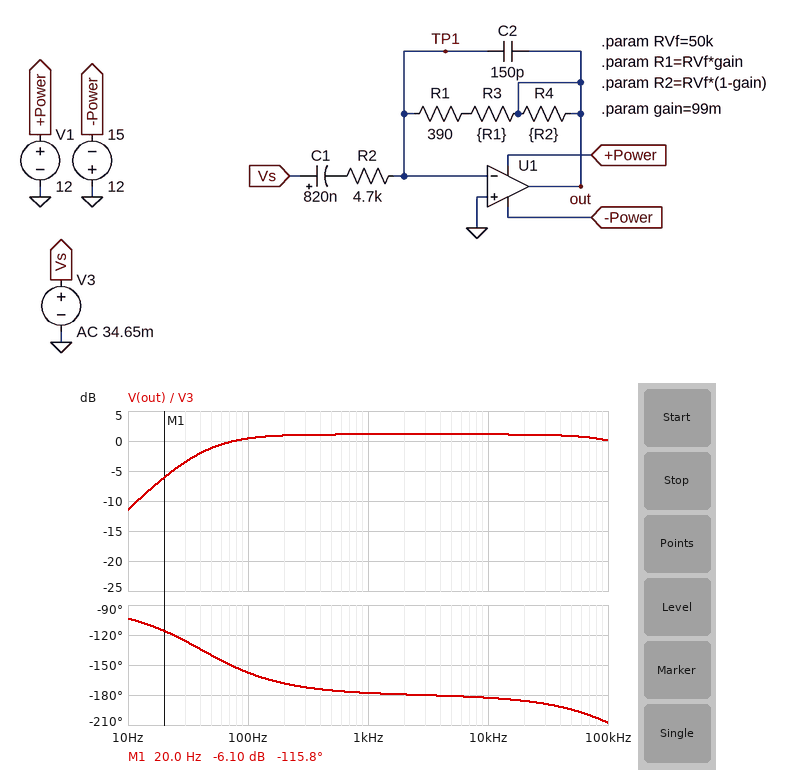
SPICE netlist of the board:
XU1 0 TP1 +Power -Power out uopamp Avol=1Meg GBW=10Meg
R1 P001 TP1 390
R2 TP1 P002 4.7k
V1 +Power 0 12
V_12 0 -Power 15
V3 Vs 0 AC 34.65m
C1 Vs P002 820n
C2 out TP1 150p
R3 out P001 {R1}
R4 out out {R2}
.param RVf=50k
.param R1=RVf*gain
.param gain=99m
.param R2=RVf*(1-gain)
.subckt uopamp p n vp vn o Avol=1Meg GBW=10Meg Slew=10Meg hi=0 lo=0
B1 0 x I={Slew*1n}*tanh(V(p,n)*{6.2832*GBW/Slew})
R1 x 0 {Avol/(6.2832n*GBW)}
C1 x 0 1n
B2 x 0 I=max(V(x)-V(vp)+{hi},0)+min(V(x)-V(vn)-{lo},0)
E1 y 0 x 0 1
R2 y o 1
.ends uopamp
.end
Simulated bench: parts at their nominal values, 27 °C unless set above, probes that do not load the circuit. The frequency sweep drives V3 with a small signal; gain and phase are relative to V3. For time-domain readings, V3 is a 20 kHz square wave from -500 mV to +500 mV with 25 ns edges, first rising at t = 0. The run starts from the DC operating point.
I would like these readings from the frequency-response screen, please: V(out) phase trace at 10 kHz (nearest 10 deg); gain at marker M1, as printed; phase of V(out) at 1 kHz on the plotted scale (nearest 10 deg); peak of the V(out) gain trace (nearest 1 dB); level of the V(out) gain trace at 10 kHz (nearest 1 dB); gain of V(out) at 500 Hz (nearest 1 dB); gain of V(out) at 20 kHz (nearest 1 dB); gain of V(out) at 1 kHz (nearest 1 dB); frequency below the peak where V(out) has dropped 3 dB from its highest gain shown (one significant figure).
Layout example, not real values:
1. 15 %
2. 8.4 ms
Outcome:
1. -180 deg
2. -6.10 dB
3. -180 deg
4. 1 dB
5. 1 dB
6. 1 dB
7. 1 dB
8. 1 dB
9. 40 Hz
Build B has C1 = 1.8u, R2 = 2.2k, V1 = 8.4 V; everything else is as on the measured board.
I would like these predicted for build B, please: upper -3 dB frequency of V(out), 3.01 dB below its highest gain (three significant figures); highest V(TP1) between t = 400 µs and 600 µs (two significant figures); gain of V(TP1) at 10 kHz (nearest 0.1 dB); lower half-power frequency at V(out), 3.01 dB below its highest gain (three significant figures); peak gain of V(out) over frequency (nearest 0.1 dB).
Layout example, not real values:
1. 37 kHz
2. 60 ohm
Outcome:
1. 189 kHz
2. 44 mV
3. -52.3 dB
4. 40.2 Hz
5. 7.7 dB
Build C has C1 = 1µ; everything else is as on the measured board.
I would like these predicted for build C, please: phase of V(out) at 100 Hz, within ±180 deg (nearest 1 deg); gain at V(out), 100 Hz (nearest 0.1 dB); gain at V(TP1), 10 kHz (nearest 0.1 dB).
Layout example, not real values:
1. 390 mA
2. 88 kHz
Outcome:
1. -161 deg
2. 0.6 dB
3. -58.9 dB
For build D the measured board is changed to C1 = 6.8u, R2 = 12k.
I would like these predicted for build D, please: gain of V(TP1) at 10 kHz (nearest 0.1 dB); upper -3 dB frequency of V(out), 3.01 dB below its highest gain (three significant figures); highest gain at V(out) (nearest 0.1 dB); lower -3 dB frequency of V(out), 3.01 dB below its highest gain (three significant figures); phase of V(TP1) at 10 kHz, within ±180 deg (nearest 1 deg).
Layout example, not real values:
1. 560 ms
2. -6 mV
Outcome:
1. -67.0 dB
2. 197 kHz
3. -7.0 dB
4. 1.95 Hz
5. 87 deg
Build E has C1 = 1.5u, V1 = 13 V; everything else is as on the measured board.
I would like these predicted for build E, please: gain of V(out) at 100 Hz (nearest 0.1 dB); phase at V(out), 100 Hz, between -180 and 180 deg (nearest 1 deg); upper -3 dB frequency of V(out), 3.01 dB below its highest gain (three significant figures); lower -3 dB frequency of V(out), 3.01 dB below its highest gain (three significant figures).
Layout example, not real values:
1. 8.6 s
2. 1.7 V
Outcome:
1. 0.9 dB
2. -167 deg
3. 194 kHz
4. 22.6 Hz
